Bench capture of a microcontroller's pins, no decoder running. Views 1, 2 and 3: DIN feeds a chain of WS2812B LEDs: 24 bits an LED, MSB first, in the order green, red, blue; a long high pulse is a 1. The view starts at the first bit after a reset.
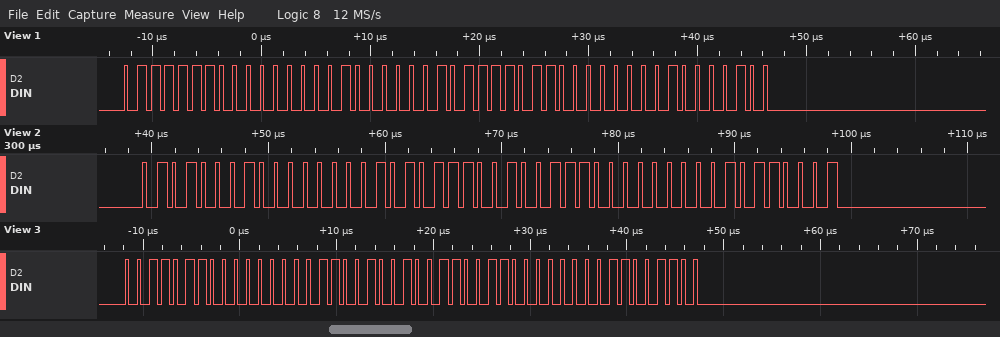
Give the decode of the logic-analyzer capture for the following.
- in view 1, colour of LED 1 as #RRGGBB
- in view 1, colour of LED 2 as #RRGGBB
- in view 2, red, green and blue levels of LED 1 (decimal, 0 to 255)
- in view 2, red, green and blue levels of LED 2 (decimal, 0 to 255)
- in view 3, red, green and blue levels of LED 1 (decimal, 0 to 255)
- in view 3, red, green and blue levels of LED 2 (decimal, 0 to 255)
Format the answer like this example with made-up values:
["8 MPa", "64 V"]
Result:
["#007E81", "#007B84", "0, 81, 174", "0, 78, 177", "0, 54, 201", "0, 51, 204"]
